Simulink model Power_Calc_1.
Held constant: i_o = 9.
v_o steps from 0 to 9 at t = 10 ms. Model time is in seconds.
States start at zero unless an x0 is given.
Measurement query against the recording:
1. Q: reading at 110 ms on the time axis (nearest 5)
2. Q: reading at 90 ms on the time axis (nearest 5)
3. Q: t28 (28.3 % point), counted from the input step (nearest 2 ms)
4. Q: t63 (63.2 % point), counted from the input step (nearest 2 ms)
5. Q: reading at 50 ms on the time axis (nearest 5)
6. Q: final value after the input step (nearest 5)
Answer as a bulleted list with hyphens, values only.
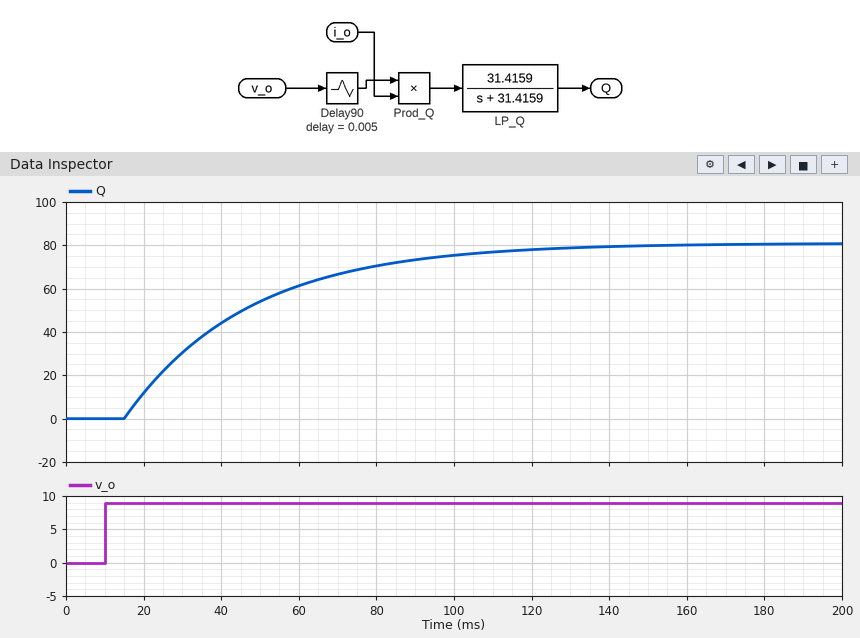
- 75
- 75
- 16 ms
- 36 ms
- 55
- 80
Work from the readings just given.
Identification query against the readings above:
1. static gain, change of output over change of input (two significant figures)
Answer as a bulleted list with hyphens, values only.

- 8.9
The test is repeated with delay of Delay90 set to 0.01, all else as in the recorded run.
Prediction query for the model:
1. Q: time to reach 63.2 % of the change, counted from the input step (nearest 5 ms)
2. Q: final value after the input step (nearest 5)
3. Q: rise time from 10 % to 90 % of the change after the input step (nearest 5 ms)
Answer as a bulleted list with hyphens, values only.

- 40 ms
- 80
- 70 ms
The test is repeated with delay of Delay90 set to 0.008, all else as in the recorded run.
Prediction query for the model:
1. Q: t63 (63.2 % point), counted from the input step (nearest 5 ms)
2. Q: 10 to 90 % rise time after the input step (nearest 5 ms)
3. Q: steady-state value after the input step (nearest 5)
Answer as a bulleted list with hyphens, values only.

- 40 ms
- 70 ms
- 80
